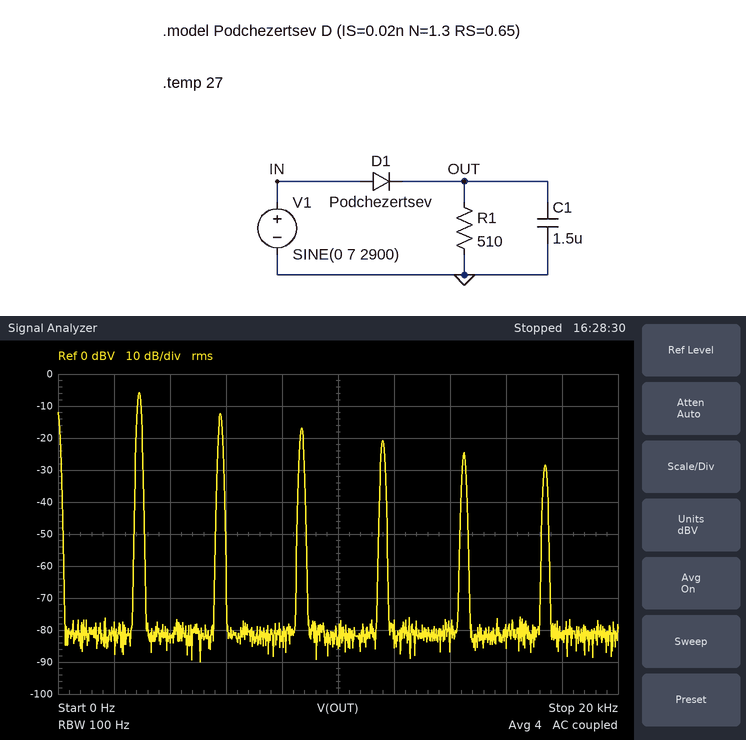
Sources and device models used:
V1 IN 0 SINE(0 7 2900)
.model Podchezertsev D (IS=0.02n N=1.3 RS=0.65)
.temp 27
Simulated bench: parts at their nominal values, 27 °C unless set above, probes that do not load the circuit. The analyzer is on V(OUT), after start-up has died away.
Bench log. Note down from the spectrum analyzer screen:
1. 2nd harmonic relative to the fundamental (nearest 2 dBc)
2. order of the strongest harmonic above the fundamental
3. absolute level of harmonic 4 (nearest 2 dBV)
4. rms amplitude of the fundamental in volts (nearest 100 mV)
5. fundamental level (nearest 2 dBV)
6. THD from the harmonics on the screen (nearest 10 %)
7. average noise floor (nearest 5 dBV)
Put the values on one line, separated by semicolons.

-6 dBc; 2; -20 dBV; 500 mV; -6 dBV; 60 %; -80 dBV
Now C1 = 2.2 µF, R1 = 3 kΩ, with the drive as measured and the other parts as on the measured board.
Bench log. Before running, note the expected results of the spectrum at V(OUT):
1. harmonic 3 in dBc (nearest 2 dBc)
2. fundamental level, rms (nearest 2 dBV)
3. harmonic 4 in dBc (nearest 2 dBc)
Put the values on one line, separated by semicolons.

-10 dBc; -22 dBV; -12 dBc
